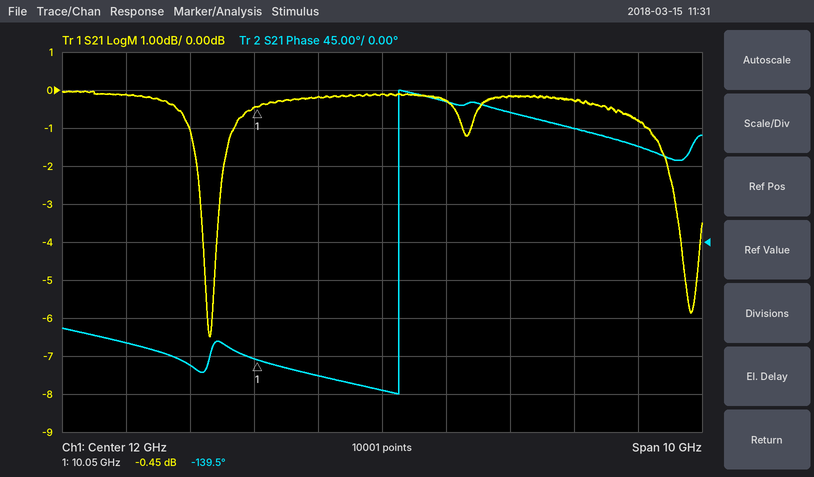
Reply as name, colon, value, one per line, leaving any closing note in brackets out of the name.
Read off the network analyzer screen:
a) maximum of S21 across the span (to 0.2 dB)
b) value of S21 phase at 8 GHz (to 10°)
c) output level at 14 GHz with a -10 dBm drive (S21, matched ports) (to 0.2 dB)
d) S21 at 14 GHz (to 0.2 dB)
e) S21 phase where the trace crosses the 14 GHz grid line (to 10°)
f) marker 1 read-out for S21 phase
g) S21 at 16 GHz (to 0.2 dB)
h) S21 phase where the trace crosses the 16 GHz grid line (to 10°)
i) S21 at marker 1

maximum of S21 across the span: 0.0 dB
value of S21 phase at 8 GHz: -120°
output level at 14 GHz with a -10 dBm drive (S21, matched ports): -10.2 dBm
S21 at 14 GHz: -0.2 dB
S21 phase where the trace crosses the 14 GHz grid line: 150°
marker 1 read-out for S21 phase: -139.5°
S21 at 16 GHz: -0.8 dB
S21 phase where the trace crosses the 16 GHz grid line: 110°
S21 at marker 1: -0.45 dB
